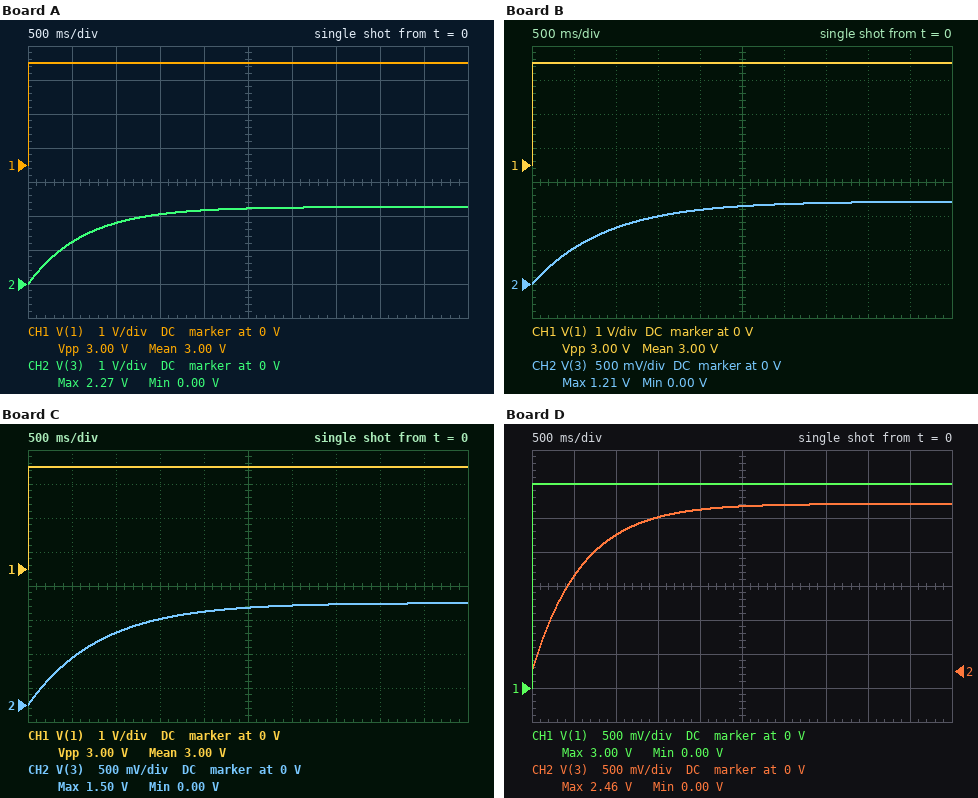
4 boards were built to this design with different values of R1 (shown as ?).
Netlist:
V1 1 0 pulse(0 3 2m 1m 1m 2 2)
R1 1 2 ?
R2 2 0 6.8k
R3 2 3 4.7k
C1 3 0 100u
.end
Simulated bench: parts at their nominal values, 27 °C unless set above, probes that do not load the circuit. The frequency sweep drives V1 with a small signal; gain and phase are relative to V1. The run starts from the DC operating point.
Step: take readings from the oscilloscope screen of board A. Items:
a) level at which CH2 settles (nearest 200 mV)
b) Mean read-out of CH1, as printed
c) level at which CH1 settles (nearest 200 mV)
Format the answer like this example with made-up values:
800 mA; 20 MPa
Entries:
2.2 V; 3.00 V; 3.0 V
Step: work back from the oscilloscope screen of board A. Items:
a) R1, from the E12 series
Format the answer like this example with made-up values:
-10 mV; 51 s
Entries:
2.2 kΩ
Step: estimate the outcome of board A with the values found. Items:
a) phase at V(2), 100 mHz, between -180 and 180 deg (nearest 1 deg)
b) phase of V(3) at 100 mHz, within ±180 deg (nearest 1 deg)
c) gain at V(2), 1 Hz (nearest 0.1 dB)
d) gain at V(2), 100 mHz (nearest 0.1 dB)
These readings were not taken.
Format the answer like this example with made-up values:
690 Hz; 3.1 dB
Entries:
-5 deg; -22 deg; -4.9 dB; -2.7 dB
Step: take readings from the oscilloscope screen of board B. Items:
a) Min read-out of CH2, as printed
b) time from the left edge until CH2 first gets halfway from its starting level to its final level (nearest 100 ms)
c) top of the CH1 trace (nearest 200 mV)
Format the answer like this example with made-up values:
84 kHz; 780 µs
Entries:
0.00 V; 600 ms; 3.0 V
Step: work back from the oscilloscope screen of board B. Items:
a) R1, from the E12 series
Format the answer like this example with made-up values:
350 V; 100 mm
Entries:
10 kΩ
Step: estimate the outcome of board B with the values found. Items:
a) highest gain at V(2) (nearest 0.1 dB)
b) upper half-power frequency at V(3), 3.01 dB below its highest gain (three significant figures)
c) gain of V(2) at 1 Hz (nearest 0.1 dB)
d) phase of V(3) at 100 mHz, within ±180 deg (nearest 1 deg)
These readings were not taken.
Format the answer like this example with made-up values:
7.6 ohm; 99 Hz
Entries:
-7.9 dB; 182 mHz; -12.9 dB; -29 deg
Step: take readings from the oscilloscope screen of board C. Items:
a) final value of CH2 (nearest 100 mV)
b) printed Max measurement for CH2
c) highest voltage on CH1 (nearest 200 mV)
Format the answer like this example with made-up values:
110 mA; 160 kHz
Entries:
1.5 V; 1.50 V; 3.0 V
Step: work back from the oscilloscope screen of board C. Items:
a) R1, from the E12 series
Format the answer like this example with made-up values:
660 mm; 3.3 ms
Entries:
6.8 kΩ
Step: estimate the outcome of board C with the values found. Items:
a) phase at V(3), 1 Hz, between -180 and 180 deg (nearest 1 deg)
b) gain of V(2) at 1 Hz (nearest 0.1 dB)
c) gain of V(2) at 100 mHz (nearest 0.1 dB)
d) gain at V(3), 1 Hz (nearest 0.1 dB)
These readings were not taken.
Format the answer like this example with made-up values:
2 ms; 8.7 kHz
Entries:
-79 deg; -10.4 dB; -6.7 dB; -20.3 dB
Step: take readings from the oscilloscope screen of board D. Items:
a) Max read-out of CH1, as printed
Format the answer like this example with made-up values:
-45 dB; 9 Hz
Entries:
3.00 V
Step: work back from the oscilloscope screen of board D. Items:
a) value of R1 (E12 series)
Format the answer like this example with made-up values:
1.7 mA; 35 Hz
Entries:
1.5 kΩ
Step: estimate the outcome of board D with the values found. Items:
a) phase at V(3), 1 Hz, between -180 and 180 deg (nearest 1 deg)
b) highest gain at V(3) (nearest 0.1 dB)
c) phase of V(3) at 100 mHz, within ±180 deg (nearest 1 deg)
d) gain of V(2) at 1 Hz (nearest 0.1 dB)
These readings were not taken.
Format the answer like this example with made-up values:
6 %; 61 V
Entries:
-75 deg; -1.7 dB; -20 deg; -3.6 dB
